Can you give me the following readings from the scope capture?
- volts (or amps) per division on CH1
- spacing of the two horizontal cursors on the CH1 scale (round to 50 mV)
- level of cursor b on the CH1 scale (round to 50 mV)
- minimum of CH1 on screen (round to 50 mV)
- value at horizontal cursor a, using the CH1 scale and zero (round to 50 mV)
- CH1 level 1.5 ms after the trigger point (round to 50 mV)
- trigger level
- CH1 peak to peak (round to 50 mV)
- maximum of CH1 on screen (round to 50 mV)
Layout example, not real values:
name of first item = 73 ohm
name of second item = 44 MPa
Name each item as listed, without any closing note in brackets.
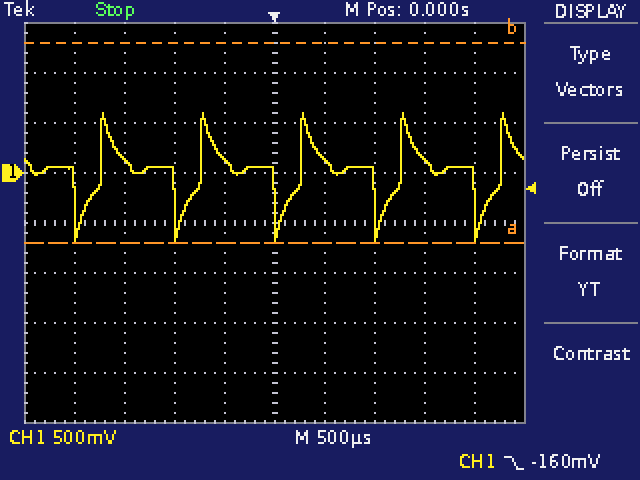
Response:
volts (or amps) per division on CH1 = 500 mV
spacing of the two horizontal cursors on the CH1 scale = 2.00 V
level of cursor b on the CH1 scale = 1.30 V
minimum of CH1 on screen = -700 mV
value at horizontal cursor a, using the CH1 scale and zero = -700 mV
CH1 level 1.5 ms after the trigger point = 150 mV
trigger level = -160 mV
CH1 peak to peak = 1.30 V
maximum of CH1 on screen = 600 mV
